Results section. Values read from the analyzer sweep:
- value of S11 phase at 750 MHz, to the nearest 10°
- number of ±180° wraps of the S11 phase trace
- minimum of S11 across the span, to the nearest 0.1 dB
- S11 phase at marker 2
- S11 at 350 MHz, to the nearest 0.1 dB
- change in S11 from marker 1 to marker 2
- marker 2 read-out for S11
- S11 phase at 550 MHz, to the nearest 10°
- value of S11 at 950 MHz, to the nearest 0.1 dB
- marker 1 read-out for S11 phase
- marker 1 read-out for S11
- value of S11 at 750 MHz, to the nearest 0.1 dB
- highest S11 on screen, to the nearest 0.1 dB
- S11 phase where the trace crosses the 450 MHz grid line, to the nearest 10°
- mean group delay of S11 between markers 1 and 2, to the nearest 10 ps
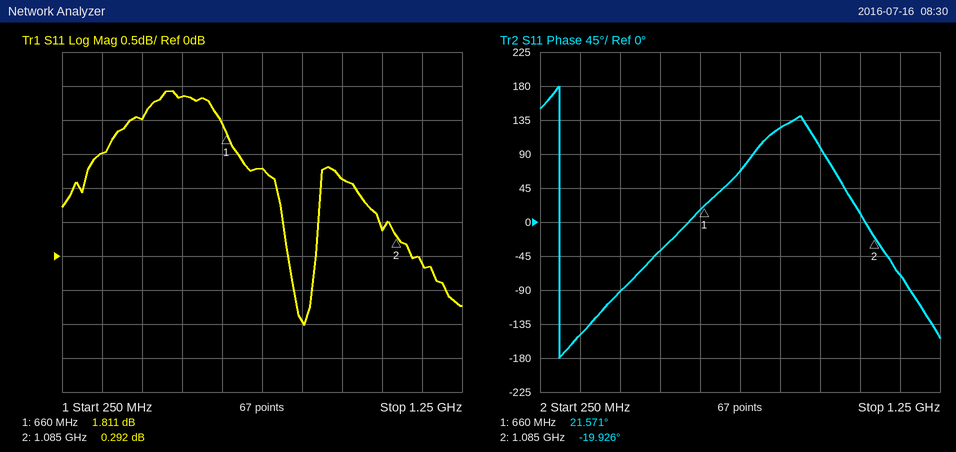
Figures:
70°
1
-1.0 dB
-19.926°
1.5 dB
-1.519 dB
0.292 dB
-40°
1.1 dB
21.571°
1.811 dB
1.3 dB
2.4 dB
-90°
270 ps
